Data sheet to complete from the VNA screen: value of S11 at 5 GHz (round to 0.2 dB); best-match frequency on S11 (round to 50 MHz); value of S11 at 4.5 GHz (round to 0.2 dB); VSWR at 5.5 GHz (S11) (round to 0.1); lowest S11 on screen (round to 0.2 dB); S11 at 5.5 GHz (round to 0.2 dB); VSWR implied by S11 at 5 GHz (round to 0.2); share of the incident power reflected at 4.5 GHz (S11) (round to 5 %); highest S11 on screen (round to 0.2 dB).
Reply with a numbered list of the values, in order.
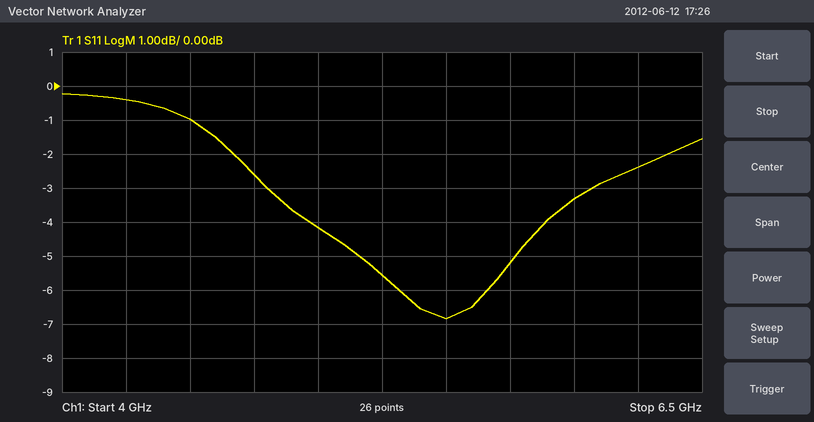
1. -4.2 dB
2. 5.50 GHz
3. -1.0 dB
4. 2.7
5. -6.8 dB
6. -6.8 dB
7. 4.2
8. 80 %
9. -0.2 dB
